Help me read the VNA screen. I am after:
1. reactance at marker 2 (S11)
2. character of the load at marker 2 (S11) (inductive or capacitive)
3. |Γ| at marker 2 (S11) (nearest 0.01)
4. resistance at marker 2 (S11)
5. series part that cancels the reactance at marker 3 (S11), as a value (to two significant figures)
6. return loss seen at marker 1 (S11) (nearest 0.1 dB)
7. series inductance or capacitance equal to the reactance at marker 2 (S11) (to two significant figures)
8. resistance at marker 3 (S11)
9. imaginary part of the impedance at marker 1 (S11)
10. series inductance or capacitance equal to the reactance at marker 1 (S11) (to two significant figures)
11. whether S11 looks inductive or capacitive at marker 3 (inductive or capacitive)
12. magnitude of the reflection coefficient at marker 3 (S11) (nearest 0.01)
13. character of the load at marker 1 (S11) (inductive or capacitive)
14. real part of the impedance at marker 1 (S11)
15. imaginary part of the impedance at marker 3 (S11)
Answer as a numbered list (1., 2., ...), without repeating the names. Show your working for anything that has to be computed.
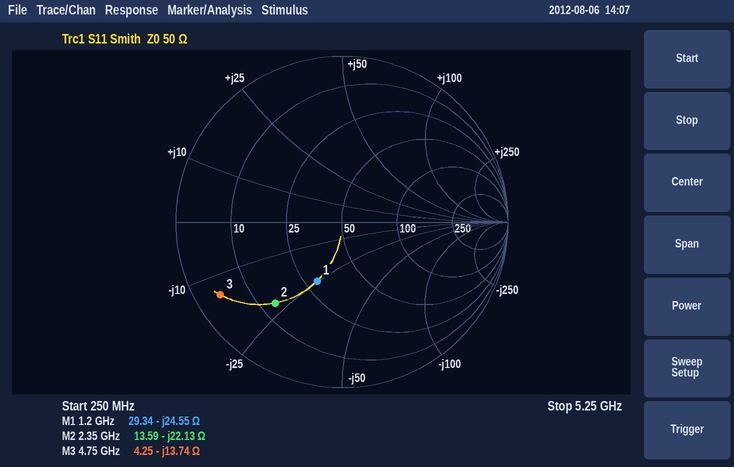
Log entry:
1. -22.13 Ω
2. capacitive
3. 0.63
4. 13.59 Ω
5. L = 13.74 Ω/(2π × 4.75 GHz) ≈ 460 pH
6. 8.3 dB
7. C = 1/(2π × 2.35 GHz × 22.13 Ω) ≈ 3.1 pF
8. 4.25 Ω
9. -24.55 Ω
10. C = 1/(2π × 1.2 GHz × 24.55 Ω) ≈ 5.4 pF
11. capacitive
12. 0.85
13. capacitive
14. 29.34 Ω
15. -13.74 Ω
